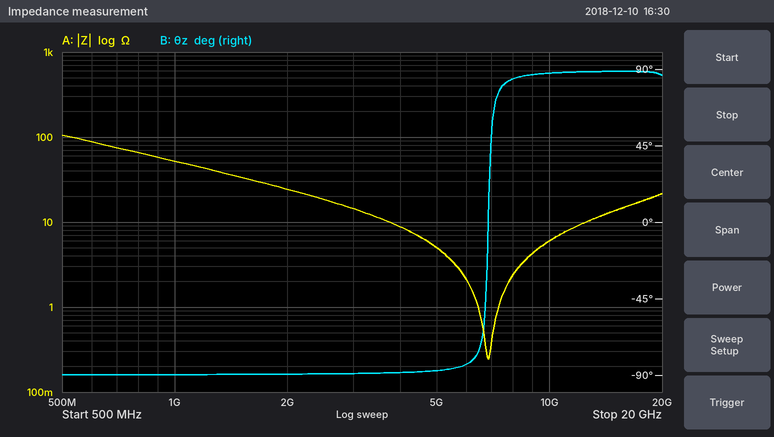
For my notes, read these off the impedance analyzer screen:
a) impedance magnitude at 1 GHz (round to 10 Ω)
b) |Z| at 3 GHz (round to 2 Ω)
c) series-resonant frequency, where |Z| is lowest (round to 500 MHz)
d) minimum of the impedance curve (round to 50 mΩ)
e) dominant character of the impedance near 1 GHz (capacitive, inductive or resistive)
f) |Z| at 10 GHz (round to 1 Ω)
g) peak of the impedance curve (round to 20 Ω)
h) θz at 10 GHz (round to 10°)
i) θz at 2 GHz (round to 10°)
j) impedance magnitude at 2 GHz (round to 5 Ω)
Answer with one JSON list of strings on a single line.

["50 Ω", "14 Ω", "7.0 GHz", "250 mΩ", "capacitive", "6 Ω", "100 Ω", "90°", "-90°", "25 Ω"]
